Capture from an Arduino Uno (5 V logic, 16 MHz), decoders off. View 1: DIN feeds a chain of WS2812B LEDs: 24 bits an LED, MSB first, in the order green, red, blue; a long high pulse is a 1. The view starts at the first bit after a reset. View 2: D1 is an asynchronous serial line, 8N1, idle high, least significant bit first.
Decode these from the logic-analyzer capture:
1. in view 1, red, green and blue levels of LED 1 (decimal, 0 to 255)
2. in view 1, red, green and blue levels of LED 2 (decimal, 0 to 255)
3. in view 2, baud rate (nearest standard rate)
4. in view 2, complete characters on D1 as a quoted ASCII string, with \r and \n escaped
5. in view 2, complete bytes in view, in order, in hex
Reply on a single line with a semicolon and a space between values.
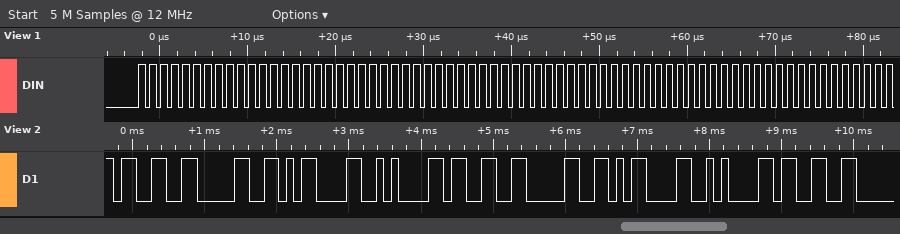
255, 255, 255; 255, 255, 255; 9600 baud; "30\r\n30\r\n3"; 0x33 0x30 0x0D 0x0A 0x33 0x30 0x0D 0x0A 0x33
